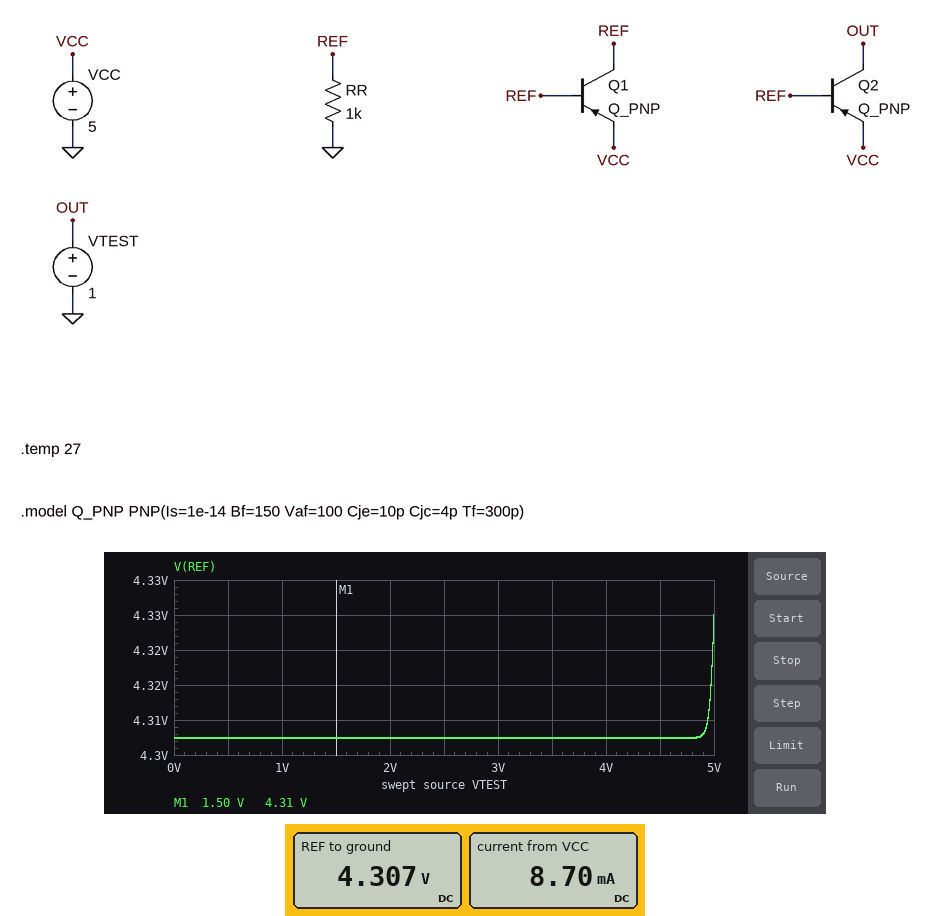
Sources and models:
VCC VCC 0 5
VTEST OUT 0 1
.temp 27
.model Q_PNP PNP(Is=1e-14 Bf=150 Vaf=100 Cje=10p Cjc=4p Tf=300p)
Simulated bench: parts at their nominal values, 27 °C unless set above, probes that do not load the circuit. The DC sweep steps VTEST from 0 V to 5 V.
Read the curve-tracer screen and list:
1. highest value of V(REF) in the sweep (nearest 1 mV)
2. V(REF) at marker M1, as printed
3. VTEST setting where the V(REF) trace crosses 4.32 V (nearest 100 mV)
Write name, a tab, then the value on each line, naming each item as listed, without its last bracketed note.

highest value of V(REF) in the sweep	4.325 V
V(REF) at marker M1, as printed	4.31 V
VTEST setting where the V(REF) trace crosses 4.32 V	5.0 V
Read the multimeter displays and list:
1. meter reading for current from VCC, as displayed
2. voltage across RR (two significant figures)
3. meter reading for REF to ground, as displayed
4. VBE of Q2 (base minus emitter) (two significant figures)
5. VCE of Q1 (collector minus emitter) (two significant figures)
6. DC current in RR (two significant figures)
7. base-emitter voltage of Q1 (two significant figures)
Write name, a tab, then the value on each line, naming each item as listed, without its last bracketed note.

meter reading for current from VCC, as displayed	8.70 mA
voltage across RR	4.3 V
meter reading for REF to ground, as displayed	4.307 V
VBE of Q2 (base minus emitter)	-690 mV
VCE of Q1 (collector minus emitter)	-690 mV
DC current in RR	4.3 mA
base-emitter voltage of Q1	-690 mV
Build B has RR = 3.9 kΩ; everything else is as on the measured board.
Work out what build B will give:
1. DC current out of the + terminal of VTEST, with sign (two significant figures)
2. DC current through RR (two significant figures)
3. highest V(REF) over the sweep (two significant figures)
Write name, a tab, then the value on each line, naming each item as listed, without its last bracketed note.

DC current out of the + terminal of VTEST, with sign	-1.1 mA
DC current through RR	1.1 mA
highest V(REF) over the sweep	4.4 V
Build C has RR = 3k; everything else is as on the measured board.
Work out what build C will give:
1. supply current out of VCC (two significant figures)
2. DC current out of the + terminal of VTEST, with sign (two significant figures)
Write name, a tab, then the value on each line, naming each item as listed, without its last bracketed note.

supply current out of VCC	2.9 mA
DC current out of the + terminal of VTEST, with sign	-1.5 mA
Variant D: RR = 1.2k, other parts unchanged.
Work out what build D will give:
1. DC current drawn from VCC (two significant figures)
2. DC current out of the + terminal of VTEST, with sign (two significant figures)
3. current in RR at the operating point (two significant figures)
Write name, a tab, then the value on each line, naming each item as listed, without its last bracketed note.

DC current drawn from VCC	7.3 mA
DC current out of the + terminal of VTEST, with sign	-3.7 mA
current in RR at the operating point	3.6 mA
